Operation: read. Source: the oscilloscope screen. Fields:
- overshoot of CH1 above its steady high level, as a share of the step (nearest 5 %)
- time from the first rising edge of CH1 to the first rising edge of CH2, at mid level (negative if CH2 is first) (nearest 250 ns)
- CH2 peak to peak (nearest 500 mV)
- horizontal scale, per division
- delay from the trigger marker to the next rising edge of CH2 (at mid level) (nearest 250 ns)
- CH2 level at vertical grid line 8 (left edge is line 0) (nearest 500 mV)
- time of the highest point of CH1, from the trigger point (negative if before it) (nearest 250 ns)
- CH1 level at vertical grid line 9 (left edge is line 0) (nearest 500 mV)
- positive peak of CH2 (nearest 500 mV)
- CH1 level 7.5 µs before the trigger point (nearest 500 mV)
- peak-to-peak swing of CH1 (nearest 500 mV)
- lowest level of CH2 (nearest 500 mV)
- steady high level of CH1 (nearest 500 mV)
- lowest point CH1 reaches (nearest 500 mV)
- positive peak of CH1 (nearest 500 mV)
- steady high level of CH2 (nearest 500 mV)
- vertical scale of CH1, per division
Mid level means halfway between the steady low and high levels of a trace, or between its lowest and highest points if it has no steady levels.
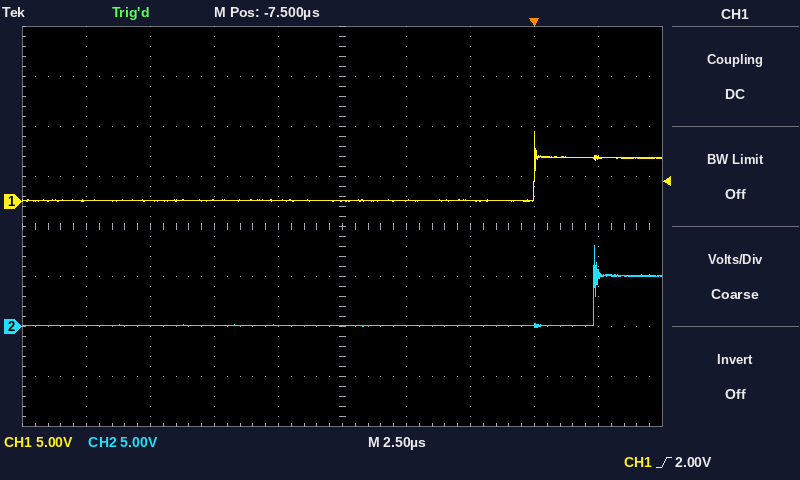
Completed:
60 %
+2.25 µs
8.0 V
2.5 µs
2.25 µs
0.0 V
0.00 µs
4.5 V
8.0 V
0.0 V
7.0 V
0.0 V
4.5 V
0.0 V
7.0 V
5.0 V
5 V
